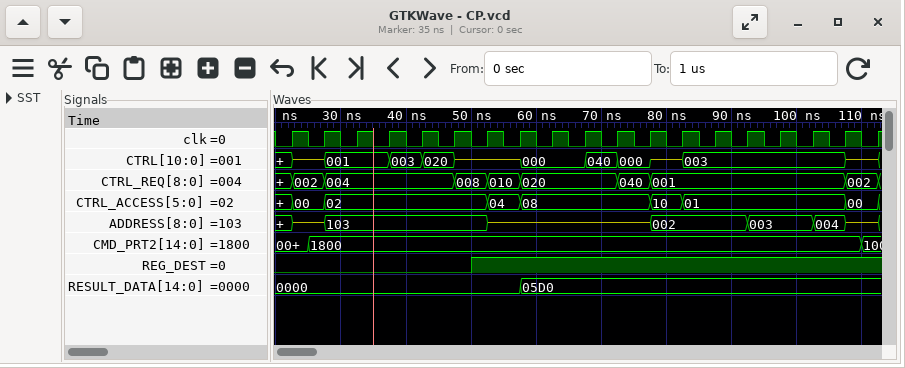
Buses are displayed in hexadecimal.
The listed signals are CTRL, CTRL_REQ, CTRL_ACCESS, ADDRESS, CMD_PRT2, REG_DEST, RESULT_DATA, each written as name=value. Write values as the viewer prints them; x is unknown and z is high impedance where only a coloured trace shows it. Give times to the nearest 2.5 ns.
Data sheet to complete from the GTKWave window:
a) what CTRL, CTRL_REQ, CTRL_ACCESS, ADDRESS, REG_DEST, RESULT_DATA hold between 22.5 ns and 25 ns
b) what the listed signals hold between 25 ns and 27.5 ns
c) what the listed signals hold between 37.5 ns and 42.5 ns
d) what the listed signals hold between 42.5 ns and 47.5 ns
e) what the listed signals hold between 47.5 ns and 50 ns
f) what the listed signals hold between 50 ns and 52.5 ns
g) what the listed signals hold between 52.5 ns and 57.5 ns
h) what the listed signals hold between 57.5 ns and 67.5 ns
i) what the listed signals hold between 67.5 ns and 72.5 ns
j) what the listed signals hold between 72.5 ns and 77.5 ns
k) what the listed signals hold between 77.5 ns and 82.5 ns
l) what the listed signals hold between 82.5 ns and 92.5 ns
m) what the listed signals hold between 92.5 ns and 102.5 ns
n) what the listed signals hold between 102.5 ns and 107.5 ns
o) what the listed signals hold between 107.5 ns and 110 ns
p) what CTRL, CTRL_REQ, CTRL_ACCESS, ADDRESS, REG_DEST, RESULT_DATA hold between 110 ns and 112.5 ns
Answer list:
CTRL=z, CTRL_REQ=002, CTRL_ACCESS=00, ADDRESS=z, REG_DEST=0, RESULT_DATA=0000
CTRL=z, CTRL_REQ=002, CTRL_ACCESS=00, ADDRESS=z, CMD_PRT2=1800, REG_DEST=0, RESULT_DATA=0000
CTRL=003, CTRL_REQ=004, CTRL_ACCESS=02, ADDRESS=103, CMD_PRT2=1800, REG_DEST=0, RESULT_DATA=0000
CTRL=020, CTRL_REQ=004, CTRL_ACCESS=02, ADDRESS=103, CMD_PRT2=1800, REG_DEST=0, RESULT_DATA=0000
CTRL=z, CTRL_REQ=008, CTRL_ACCESS=02, ADDRESS=103, CMD_PRT2=1800, REG_DEST=0, RESULT_DATA=0000
CTRL=z, CTRL_REQ=008, CTRL_ACCESS=02, ADDRESS=103, CMD_PRT2=1800, REG_DEST=1, RESULT_DATA=0000
CTRL=z, CTRL_REQ=010, CTRL_ACCESS=04, ADDRESS=z, CMD_PRT2=1800, REG_DEST=1, RESULT_DATA=0000
CTRL=000, CTRL_REQ=020, CTRL_ACCESS=08, ADDRESS=z, CMD_PRT2=1800, REG_DEST=1, RESULT_DATA=05D0
CTRL=040, CTRL_REQ=020, CTRL_ACCESS=08, ADDRESS=z, CMD_PRT2=1800, REG_DEST=1, RESULT_DATA=05D0
CTRL=000, CTRL_REQ=040, CTRL_ACCESS=08, ADDRESS=z, CMD_PRT2=1800, REG_DEST=1, RESULT_DATA=05D0
CTRL=z, CTRL_REQ=001, CTRL_ACCESS=10, ADDRESS=002, CMD_PRT2=1800, REG_DEST=1, RESULT_DATA=05D0
CTRL=003, CTRL_REQ=001, CTRL_ACCESS=01, ADDRESS=002, CMD_PRT2=1800, REG_DEST=1, RESULT_DATA=05D0
CTRL=003, CTRL_REQ=001, CTRL_ACCESS=01, ADDRESS=003, CMD_PRT2=1800, REG_DEST=1, RESULT_DATA=05D0
CTRL=003, CTRL_REQ=001, CTRL_ACCESS=01, ADDRESS=004, CMD_PRT2=1800, REG_DEST=1, RESULT_DATA=05D0
CTRL=z, CTRL_REQ=002, CTRL_ACCESS=00, ADDRESS=z, CMD_PRT2=1800, REG_DEST=1, RESULT_DATA=05D0
CTRL=z, CTRL_REQ=002, CTRL_ACCESS=00, ADDRESS=z, REG_DEST=1, RESULT_DATA=05D0
